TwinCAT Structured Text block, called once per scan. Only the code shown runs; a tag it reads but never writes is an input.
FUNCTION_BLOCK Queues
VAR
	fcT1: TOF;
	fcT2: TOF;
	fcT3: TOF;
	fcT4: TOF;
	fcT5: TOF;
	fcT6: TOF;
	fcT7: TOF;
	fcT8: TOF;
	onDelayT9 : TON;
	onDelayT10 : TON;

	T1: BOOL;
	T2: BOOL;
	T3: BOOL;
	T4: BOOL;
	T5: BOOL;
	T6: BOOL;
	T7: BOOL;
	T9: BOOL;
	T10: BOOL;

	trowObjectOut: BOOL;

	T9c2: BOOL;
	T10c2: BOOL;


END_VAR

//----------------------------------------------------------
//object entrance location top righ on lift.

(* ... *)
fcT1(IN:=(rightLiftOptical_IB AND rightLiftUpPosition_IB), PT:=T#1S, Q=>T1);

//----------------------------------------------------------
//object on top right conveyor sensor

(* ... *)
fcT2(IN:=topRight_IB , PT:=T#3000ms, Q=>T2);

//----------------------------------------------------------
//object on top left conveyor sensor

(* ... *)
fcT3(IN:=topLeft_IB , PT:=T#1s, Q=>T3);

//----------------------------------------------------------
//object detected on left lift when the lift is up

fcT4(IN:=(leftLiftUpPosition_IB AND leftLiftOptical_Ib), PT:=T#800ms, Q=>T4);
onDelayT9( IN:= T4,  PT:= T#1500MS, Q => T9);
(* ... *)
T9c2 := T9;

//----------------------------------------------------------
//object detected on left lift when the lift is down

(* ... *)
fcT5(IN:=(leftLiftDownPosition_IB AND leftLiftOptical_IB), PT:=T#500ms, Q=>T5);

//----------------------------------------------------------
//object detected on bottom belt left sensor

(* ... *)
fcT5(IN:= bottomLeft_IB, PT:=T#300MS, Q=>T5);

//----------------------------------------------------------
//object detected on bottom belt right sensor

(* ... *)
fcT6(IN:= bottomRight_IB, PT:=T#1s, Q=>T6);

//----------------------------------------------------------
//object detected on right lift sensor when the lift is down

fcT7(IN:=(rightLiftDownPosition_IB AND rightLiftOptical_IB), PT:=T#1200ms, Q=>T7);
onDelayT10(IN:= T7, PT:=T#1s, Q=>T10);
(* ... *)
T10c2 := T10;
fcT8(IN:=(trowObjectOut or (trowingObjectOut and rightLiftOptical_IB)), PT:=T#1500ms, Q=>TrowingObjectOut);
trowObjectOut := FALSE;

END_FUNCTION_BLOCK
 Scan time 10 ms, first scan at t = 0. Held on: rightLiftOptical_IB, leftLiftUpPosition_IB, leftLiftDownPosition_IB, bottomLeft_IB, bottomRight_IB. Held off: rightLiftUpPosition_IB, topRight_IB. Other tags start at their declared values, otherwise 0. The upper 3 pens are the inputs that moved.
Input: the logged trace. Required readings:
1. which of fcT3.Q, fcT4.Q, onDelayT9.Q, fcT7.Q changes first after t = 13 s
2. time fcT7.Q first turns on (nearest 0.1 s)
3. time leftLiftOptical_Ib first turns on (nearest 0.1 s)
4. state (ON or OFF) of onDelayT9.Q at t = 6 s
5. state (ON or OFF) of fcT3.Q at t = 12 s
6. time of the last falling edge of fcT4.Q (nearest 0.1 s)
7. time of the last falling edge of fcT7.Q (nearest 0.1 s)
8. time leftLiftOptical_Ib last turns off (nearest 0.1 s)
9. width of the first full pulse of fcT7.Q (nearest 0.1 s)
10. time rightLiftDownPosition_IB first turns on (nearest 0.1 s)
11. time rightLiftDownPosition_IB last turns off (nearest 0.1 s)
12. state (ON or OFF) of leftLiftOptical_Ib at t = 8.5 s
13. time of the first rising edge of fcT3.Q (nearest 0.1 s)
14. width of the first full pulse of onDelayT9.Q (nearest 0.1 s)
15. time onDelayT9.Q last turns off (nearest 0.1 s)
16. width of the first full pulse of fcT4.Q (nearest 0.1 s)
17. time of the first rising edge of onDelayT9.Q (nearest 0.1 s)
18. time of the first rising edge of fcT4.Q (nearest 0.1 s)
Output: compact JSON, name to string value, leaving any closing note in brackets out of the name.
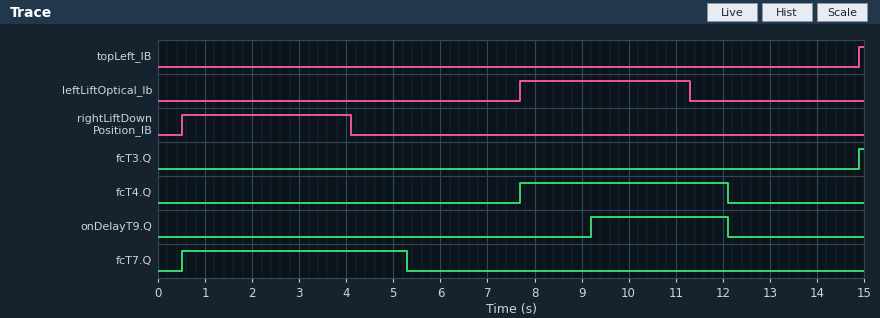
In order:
{"which of fcT3.Q, fcT4.Q, onDelayT9.Q, fcT7.Q changes first after t = 13 s": "fcT3.Q", "time fcT7.Q first turns on": "0.5 s", "time leftLiftOptical_Ib first turns on": "7.7 s", "state (ON or OFF) of onDelayT9.Q at t = 6 s": "OFF", "state (ON or OFF) of fcT3.Q at t = 12 s": "OFF", "time of the last falling edge of fcT4.Q": "12.1 s", "time of the last falling edge of fcT7.Q": "5.3 s", "time leftLiftOptical_Ib last turns off": "11.3 s", "width of the first full pulse of fcT7.Q": "4.8 s", "time rightLiftDownPosition_IB first turns on": "0.5 s", "time rightLiftDownPosition_IB last turns off": "4.1 s", "state (ON or OFF) of leftLiftOptical_Ib at t = 8.5 s": "ON", "time of the first rising edge of fcT3.Q": "14.9 s", "width of the first full pulse of onDelayT9.Q": "2.9 s", "time onDelayT9.Q last turns off": "12.1 s", "width of the first full pulse of fcT4.Q": "4.4 s", "time of the first rising edge of onDelayT9.Q": "9.2 s", "time of the first rising edge of fcT4.Q": "7.7 s"}
